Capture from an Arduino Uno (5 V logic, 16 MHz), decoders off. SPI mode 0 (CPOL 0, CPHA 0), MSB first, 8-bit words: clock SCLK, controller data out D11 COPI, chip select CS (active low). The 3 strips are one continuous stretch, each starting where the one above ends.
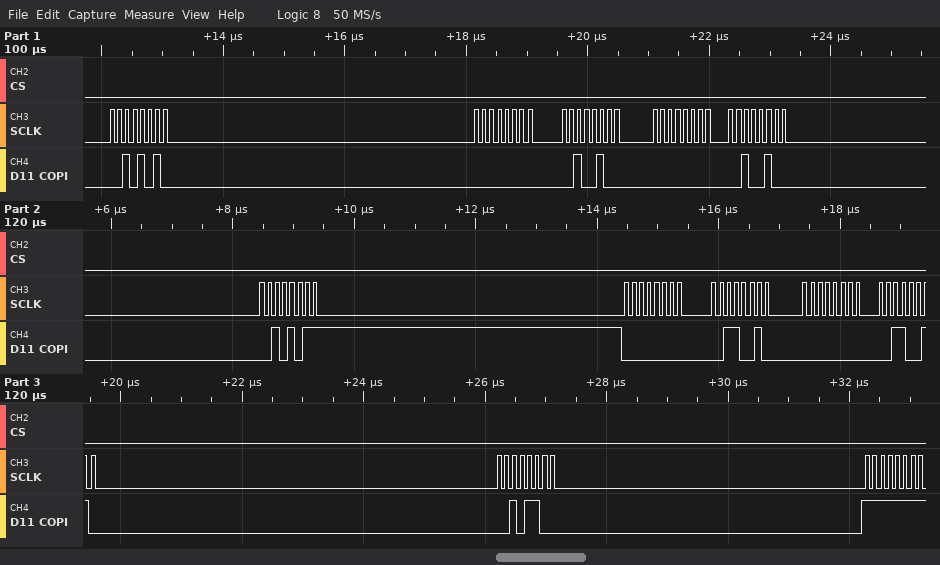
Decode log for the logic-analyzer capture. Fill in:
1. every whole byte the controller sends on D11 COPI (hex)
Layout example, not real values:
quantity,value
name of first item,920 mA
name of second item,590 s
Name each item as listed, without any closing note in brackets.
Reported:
quantity,value
every whole byte the controller sends on D11 COPI,2A 00 24 00 24 2B 00 32 00 32 2C FF
